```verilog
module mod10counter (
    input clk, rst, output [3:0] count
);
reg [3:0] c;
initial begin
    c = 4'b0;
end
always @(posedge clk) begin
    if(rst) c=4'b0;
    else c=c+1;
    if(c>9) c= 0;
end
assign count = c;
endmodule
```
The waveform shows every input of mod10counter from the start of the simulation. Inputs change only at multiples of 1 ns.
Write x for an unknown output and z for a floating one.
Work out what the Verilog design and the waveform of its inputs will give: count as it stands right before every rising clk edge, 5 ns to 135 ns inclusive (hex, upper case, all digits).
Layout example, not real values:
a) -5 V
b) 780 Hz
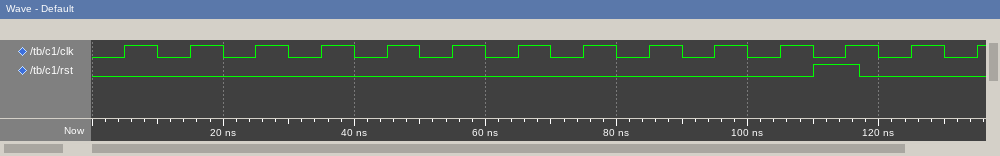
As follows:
a) 0, 1, 2, 3, 4, 5, 6, 7, 8, 9, 0, 1, 0, 1
